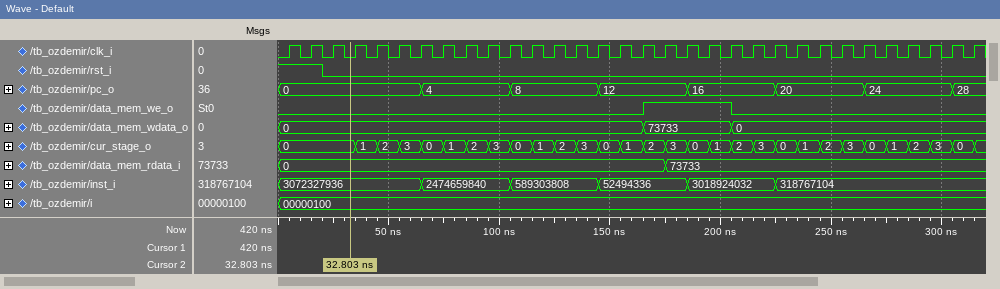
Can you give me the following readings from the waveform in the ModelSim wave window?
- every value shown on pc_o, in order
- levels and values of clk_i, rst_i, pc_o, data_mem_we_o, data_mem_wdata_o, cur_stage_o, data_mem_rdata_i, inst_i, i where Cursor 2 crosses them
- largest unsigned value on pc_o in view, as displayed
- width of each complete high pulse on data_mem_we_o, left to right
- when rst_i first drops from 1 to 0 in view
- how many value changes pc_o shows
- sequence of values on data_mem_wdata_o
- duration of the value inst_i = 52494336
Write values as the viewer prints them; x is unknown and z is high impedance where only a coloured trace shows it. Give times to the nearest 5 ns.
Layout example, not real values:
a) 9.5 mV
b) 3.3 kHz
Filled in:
a) 0, 4, 8, 12, 16, 20, 24, 28
b) clk_i=0, rst_i=0, pc_o=0, data_mem_we_o=0, data_mem_wdata_o=0, cur_stage_o=0, data_mem_rdata_i=0, inst_i=3072327936, i=00000100
c) 28
d) 40 ns
e) 20 ns
f) 7
g) 0, 73733, 0
h) 40 ns
